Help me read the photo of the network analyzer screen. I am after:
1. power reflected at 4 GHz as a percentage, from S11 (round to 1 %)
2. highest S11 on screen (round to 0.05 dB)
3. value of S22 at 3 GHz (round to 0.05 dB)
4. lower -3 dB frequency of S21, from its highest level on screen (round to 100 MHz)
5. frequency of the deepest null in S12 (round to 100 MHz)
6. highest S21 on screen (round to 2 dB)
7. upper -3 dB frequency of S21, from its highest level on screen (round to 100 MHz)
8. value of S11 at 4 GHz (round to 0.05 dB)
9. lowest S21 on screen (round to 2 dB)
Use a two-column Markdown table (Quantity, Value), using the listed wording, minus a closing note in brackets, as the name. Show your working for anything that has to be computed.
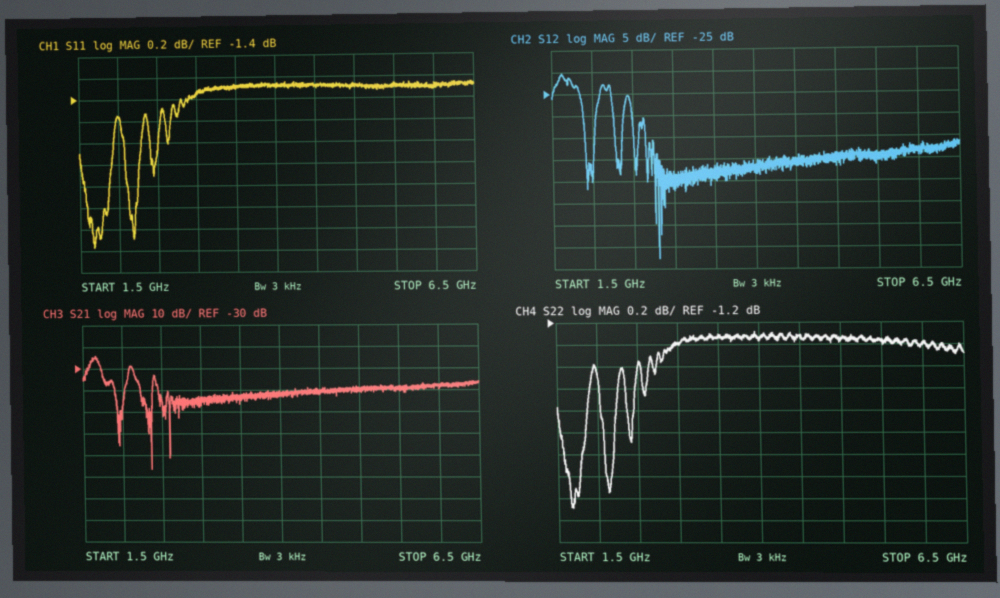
| Quantity | Value |
|---|---|
| power reflected at 4 GHz as a percentage, from S11 | 10^(-1.3/10) ≈ 74 % |
| highest S11 on screen | -1.25 dB |
| value of S22 at 3 GHz | -1.40 dB |
| lower -3 dB frequency of S21, from its highest level on screen | 1.6 GHz |
| frequency of the deepest null in S12 | 2.8 GHz |
| highest S21 on screen | -24 dB |
| upper -3 dB frequency of S21, from its highest level on screen | 1.7 GHz |
| value of S11 at 4 GHz | -1.30 dB |
| lowest S21 on screen | -76 dB |
